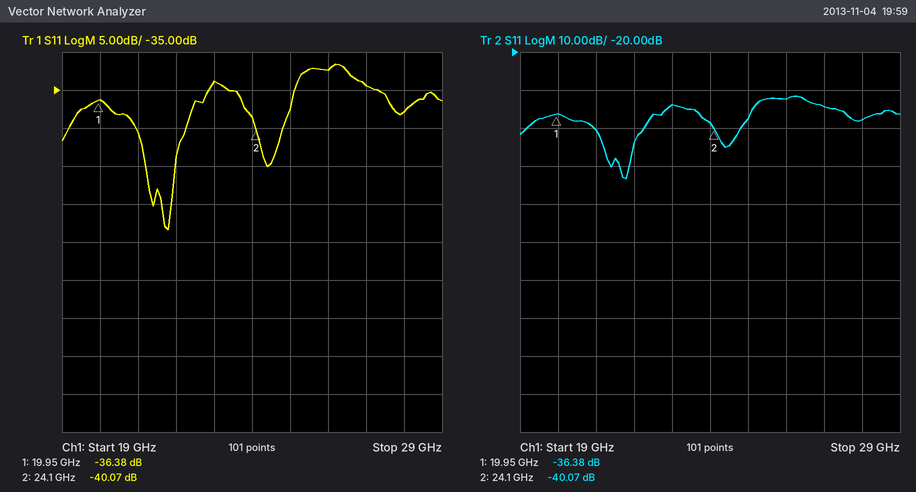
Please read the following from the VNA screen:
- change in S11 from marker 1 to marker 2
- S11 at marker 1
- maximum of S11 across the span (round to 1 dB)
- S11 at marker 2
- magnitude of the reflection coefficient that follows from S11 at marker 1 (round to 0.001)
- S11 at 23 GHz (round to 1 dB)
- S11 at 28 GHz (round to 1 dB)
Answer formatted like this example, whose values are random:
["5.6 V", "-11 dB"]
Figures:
["-3.69 dB", "-36.38 dB", "-32 dB", "-40.07 dB", "0.015", "-34 dB", "-38 dB"]
